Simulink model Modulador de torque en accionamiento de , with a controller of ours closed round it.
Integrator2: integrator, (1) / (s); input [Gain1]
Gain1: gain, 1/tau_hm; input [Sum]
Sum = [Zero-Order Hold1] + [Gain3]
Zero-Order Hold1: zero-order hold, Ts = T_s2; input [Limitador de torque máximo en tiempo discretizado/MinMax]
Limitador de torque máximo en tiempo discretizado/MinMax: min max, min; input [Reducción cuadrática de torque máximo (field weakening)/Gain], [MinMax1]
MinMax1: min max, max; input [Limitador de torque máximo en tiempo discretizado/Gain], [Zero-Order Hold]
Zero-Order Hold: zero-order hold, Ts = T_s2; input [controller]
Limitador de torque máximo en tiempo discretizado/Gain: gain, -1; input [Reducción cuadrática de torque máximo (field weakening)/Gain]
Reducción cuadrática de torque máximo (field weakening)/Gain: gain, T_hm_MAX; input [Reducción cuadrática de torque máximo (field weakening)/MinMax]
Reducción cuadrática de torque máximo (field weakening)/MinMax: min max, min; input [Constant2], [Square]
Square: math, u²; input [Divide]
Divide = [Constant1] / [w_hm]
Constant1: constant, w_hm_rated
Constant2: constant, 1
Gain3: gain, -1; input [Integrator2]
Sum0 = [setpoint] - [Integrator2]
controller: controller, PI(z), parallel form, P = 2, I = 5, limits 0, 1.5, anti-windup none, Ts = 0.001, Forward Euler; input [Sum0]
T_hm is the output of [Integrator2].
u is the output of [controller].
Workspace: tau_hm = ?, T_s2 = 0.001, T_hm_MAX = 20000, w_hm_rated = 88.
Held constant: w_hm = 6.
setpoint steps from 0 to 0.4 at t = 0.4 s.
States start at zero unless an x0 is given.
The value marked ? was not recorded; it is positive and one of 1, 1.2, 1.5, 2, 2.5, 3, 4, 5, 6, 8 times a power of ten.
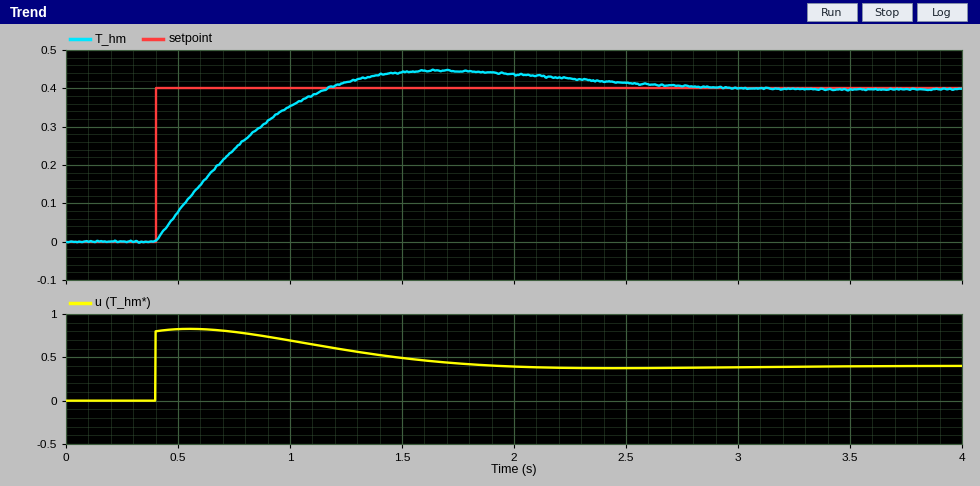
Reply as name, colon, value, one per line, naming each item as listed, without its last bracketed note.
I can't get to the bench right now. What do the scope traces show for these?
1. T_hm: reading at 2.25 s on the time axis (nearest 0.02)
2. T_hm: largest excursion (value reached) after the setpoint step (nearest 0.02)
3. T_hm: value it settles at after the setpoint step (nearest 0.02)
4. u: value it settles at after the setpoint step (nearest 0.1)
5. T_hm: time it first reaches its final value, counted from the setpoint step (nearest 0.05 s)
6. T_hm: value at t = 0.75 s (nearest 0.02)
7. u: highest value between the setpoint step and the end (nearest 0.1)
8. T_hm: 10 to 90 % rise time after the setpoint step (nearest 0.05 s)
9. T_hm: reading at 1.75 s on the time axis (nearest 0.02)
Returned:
T_hm: reading at 2.25 s on the time axis: 0.42
T_hm: largest excursion (value reached) after the setpoint step: 0.44
T_hm: value it settles at after the setpoint step: 0.40
u: value it settles at after the setpoint step: 0.4
T_hm: time it first reaches its final value, counted from the setpoint step: 0.75 s
T_hm: value at t = 0.75 s: 0.24
u: highest value between the setpoint step and the end: 0.8
T_hm: 10 to 90 % rise time after the setpoint step: 0.55 s
T_hm: reading at 1.75 s on the time axis: 0.44
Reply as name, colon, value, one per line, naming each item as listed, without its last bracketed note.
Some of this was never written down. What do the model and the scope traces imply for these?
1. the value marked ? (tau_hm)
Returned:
the value marked ?: 1
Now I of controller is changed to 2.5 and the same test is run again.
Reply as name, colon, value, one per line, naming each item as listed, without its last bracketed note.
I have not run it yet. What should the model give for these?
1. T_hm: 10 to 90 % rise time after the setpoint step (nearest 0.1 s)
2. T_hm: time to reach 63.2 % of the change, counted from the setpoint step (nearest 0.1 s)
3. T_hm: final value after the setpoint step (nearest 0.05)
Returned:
T_hm: 10 to 90 % rise time after the setpoint step: 0.9 s
T_hm: time to reach 63.2 % of the change, counted from the setpoint step: 0.5 s
T_hm: final value after the setpoint step: 0.40
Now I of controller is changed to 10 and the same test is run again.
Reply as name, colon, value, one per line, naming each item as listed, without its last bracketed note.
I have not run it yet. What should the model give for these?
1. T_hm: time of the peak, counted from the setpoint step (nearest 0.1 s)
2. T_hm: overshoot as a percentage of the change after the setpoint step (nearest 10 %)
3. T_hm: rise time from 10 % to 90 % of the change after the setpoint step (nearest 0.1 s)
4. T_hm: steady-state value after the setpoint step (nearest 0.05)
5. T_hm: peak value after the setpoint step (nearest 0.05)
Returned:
T_hm: time of the peak, counted from the setpoint step: 0.9 s
T_hm: overshoot as a percentage of the change after the setpoint step: 20 %
T_hm: rise time from 10 % to 90 % of the change after the setpoint step: 0.4 s
T_hm: steady-state value after the setpoint step: 0.40
T_hm: peak value after the setpoint step: 0.50
